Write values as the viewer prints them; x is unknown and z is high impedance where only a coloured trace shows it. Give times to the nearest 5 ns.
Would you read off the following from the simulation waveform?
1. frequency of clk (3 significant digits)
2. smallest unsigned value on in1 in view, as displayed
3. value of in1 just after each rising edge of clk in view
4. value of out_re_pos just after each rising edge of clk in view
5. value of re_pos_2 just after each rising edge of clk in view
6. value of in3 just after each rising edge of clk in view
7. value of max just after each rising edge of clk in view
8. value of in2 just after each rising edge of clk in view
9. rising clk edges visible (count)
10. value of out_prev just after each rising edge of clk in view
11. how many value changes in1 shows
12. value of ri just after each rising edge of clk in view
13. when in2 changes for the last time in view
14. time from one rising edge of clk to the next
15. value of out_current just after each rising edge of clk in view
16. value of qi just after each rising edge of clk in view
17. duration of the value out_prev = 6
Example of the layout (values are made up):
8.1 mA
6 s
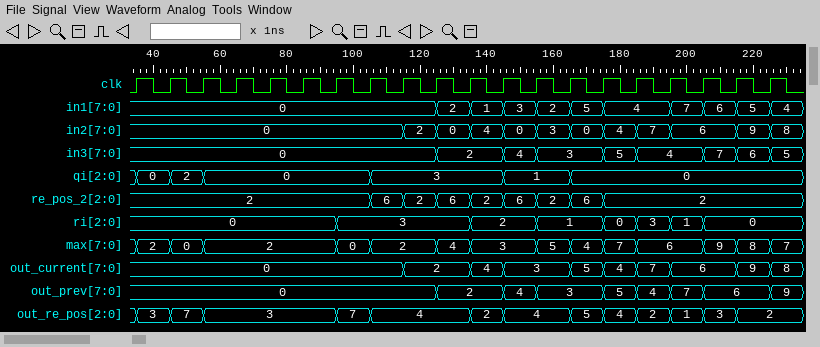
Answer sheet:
100 MHz
0
0, 0, 0, 0, 0, 0, 0, 0, 0, 2, 1, 3, 2, 5, 4, 4, 7, 6, 5, 4
3, 7, 3, 3, 3, 3, 7, 4, 4, 4, 2, 4, 4, 5, 4, 2, 1, 3, 2, 2
2, 2, 2, 2, 2, 2, 2, 6, 2, 6, 2, 6, 2, 6, 2, 2, 2, 2, 2, 2
0, 0, 0, 0, 0, 0, 0, 0, 0, 2, 2, 4, 3, 3, 5, 4, 4, 7, 6, 5
2, 0, 2, 2, 2, 2, 0, 2, 2, 4, 3, 3, 5, 4, 7, 6, 6, 9, 8, 7
0, 0, 0, 0, 0, 0, 0, 0, 2, 0, 4, 0, 3, 0, 4, 7, 6, 6, 9, 8
20
0, 0, 0, 0, 0, 0, 0, 0, 0, 2, 2, 4, 3, 3, 5, 4, 7, 6, 6, 9
10
0, 0, 0, 0, 0, 0, 3, 3, 3, 3, 2, 2, 1, 1, 0, 3, 1, 0, 0, 0
225 ns
10 ns
0, 0, 0, 0, 0, 0, 0, 0, 2, 2, 4, 3, 3, 5, 4, 7, 6, 6, 9, 8
0, 2, 0, 0, 0, 0, 0, 3, 3, 3, 3, 1, 1, 0, 0, 0, 0, 0, 0, 0
20 ns
